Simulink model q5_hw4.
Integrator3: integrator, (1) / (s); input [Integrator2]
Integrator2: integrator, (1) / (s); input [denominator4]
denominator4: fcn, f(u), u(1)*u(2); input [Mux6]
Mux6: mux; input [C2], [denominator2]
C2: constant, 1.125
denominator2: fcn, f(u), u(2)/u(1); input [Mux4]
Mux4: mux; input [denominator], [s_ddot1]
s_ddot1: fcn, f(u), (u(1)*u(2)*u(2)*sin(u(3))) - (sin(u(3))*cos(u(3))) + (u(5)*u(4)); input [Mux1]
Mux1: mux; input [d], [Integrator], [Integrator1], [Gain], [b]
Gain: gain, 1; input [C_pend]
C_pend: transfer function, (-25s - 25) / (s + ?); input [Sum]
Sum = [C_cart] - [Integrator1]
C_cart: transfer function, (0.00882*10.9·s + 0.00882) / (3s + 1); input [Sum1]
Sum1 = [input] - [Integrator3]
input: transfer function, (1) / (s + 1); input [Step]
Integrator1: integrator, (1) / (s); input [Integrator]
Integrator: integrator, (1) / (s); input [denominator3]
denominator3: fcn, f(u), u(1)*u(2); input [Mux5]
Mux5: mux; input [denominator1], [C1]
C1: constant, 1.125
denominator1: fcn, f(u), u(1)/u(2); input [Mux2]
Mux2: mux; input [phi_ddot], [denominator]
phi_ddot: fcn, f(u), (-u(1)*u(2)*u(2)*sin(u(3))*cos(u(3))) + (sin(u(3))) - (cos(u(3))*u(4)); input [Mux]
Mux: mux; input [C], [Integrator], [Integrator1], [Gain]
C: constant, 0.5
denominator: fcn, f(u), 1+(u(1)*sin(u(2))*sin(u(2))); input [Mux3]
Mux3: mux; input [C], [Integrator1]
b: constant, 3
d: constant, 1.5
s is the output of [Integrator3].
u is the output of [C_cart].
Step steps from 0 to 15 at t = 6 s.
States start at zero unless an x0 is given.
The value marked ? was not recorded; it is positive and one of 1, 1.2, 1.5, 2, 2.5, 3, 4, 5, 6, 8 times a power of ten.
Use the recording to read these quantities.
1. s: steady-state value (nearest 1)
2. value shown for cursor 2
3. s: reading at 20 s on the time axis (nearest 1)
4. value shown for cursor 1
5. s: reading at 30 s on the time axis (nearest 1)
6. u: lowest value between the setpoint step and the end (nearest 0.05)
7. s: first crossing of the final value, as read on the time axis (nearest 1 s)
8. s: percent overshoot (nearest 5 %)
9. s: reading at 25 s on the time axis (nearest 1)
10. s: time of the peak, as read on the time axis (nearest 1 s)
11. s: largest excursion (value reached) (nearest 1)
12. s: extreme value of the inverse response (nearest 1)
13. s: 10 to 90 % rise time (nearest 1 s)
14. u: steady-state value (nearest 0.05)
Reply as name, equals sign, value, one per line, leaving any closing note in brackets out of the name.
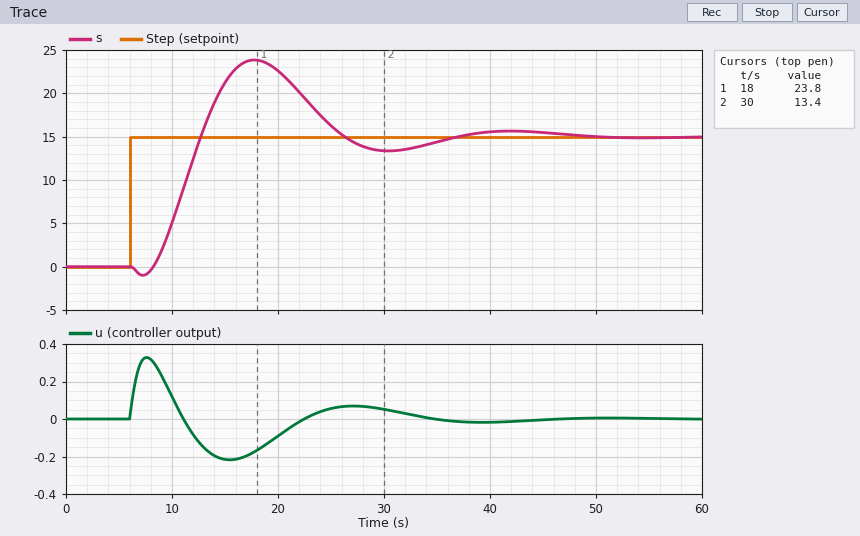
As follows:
s: steady-state value = 15
value shown for cursor 2 = 13.4
s: reading at 20 s on the time axis = 23
value shown for cursor 1 = 23.8
s: reading at 30 s on the time axis = 13
u: lowest value between the setpoint step and the end = -0.20
s: first crossing of the final value, as read on the time axis = 13 s
s: percent overshoot = 60 %
s: reading at 25 s on the time axis = 16
s: time of the peak, as read on the time axis = 18 s
s: largest excursion (value reached) = 24
s: extreme value of the inverse response = -1
s: 10 to 90 % rise time = 3 s
u: steady-state value = 0.00
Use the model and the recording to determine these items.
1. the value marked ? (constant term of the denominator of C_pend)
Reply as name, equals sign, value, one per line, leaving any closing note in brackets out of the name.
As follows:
the value marked ? = 6
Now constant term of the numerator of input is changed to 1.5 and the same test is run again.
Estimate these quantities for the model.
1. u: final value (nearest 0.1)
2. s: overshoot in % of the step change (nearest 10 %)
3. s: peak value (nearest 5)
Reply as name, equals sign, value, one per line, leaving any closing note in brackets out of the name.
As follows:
u: final value = 0.0
s: overshoot in % of the step change = 70 %
s: peak value = 40
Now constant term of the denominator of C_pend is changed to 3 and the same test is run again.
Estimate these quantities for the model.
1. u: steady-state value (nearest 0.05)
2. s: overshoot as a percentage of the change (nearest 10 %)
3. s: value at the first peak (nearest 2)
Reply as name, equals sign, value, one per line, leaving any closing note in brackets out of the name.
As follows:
u: steady-state value = 0.00
s: overshoot as a percentage of the change = 50 %
s: value at the first peak = 22
